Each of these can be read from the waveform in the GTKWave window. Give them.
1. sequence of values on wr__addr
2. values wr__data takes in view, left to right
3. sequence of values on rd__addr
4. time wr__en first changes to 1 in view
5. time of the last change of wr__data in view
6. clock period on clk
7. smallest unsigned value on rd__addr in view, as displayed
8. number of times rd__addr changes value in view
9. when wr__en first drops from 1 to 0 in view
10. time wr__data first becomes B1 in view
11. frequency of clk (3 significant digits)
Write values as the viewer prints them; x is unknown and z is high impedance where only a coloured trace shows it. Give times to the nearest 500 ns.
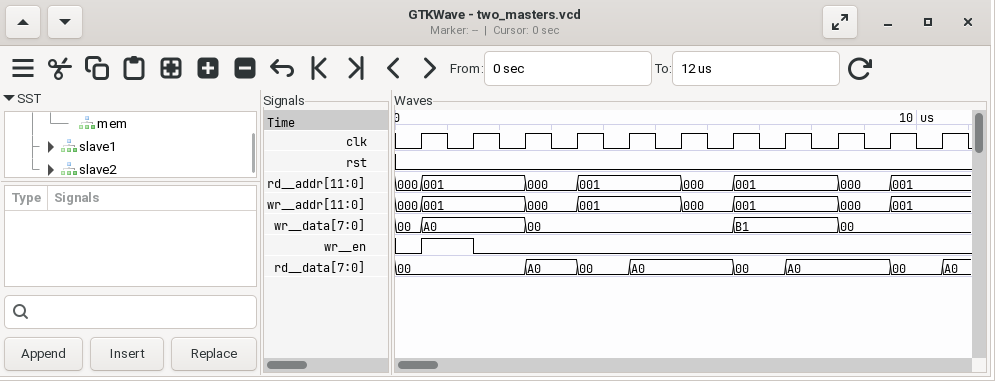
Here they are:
000, 001, 000, 001, 000, 001, 000, 001
00, A0, 00, B1, 00
000, 001, 000, 001, 000, 001, 000, 001
500 ns
8500 ns
1000 ns
000
7
1500 ns
6500 ns
1.00 MHz
